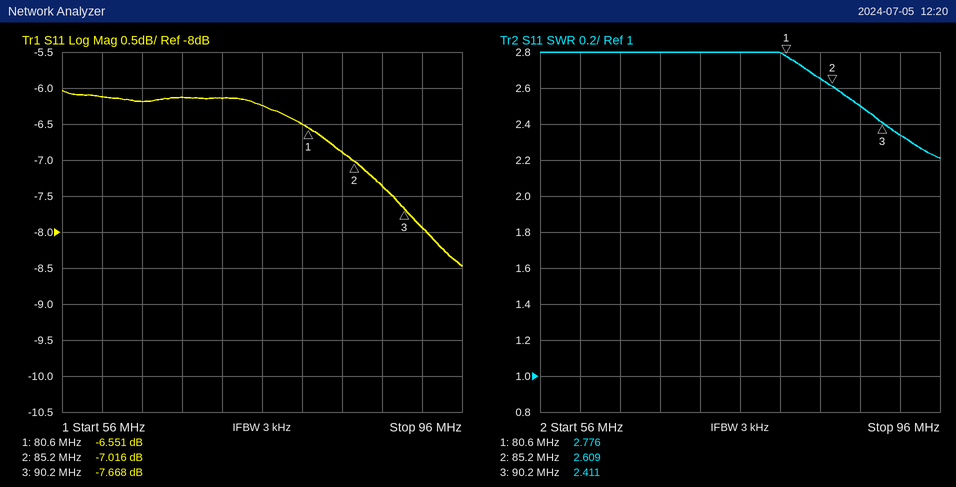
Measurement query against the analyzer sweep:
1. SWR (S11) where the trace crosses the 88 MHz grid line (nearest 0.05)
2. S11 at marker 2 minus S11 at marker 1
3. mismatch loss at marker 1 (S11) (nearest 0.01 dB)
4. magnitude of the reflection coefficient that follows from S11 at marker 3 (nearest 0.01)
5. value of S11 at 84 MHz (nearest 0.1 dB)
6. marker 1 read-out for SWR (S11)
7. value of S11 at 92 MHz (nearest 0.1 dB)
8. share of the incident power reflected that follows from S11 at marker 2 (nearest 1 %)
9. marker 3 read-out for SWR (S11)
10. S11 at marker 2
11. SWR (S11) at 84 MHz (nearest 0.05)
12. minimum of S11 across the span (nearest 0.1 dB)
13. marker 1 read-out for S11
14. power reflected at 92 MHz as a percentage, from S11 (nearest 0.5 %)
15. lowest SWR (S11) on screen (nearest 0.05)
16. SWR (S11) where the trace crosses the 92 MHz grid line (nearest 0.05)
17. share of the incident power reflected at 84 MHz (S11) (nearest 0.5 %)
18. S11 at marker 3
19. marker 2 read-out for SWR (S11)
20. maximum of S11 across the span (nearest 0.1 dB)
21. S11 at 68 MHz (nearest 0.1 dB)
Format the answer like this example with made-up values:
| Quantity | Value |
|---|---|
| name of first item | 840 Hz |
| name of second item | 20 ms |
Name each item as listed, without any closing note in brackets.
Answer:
| Quantity | Value |
|---|---|
| SWR (S11) where the trace crosses the 88 MHz grid line | 2.50 |
| S11 at marker 2 minus S11 at marker 1 | -0.465 dB |
| mismatch loss at marker 1 (S11) | 1.09 dB |
| magnitude of the reflection coefficient that follows from S11 at marker 3 | 0.41 |
| value of S11 at 84 MHz | -6.9 dB |
| marker 1 read-out for SWR | 2.776 |
| value of S11 at 92 MHz | -7.9 dB |
| share of the incident power reflected that follows from S11 at marker 2 | 20 % |
| marker 3 read-out for SWR | 2.411 |
| S11 at marker 2 | -7.016 dB |
| SWR (S11) at 84 MHz | 2.65 |
| minimum of S11 across the span | -8.5 dB |
| marker 1 read-out for S11 | -6.551 dB |
| power reflected at 92 MHz as a percentage, from S11 | 16.0 % |
| lowest SWR (S11) on screen | 2.20 |
| SWR (S11) where the trace crosses the 92 MHz grid line | 2.35 |
| share of the incident power reflected at 84 MHz (S11) | 20.5 % |
| S11 at marker 3 | -7.668 dB |
| marker 2 read-out for SWR | 2.609 |
| maximum of S11 across the span | -6.0 dB |
| S11 at 68 MHz | -6.1 dB |
